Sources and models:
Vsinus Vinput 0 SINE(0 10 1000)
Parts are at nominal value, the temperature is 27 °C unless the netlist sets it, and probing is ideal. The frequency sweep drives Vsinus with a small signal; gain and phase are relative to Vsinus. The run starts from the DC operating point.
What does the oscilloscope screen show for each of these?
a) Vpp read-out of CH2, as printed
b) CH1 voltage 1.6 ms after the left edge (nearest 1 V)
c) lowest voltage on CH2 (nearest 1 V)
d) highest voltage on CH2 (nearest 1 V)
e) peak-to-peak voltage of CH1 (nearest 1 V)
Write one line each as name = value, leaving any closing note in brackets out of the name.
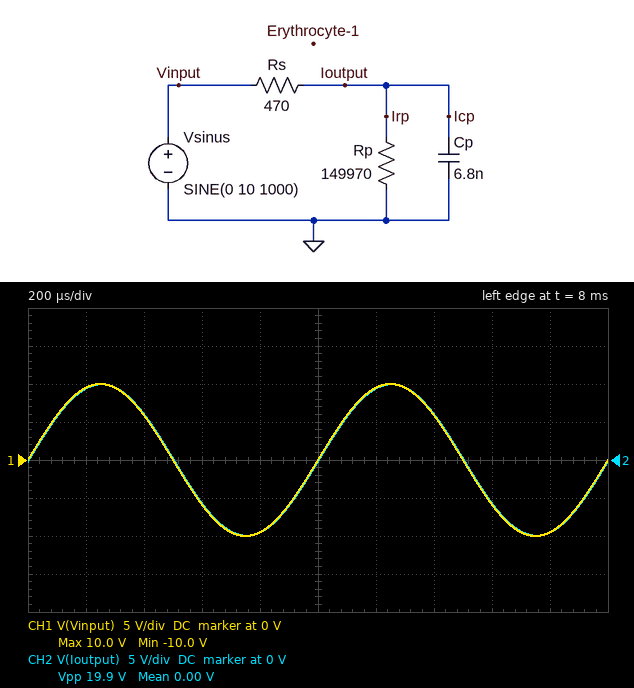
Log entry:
Vpp read-out of CH2, as printed = 19.9 V
CH1 voltage 1.6 ms after the left edge = -6 V
lowest voltage on CH2 = -10 V
highest voltage on CH2 = 10 V
peak-to-peak voltage of CH1 = 20 V
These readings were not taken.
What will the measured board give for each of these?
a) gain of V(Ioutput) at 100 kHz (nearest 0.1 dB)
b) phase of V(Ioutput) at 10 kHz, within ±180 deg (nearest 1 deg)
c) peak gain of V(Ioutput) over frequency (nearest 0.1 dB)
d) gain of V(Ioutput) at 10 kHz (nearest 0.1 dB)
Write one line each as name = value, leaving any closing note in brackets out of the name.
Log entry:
gain of V(Ioutput) at 100 kHz = -7.0 dB
phase of V(Ioutput) at 10 kHz, within ±180 deg = -11 deg
peak gain of V(Ioutput) over frequency = 0 dB
gain of V(Ioutput) at 10 kHz = -0.2 dB
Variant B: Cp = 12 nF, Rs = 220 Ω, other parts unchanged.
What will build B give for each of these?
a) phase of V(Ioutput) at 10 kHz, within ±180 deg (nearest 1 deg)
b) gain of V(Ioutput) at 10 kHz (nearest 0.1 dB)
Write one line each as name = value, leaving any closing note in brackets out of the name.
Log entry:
phase of V(Ioutput) at 10 kHz, within ±180 deg = -9 deg
gain of V(Ioutput) at 10 kHz = -0.1 dB
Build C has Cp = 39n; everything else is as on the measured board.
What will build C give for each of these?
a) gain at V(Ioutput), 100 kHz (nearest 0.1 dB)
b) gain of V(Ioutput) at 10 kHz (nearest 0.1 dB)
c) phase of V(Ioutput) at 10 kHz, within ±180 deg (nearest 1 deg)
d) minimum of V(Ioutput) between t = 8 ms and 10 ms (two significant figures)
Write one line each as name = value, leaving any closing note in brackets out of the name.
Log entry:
gain at V(Ioutput), 100 kHz = -21.3 dB
gain of V(Ioutput) at 10 kHz = -3.7 dB
phase of V(Ioutput) at 10 kHz, within ±180 deg = -49 deg
minimum of V(Ioutput) between t = 8 ms and 10 ms = -9.9 V
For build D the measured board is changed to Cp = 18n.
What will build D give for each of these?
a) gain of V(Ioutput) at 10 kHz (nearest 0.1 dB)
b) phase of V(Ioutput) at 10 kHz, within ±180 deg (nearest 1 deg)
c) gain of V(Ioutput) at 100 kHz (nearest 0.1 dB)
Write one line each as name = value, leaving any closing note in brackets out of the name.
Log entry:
gain of V(Ioutput) at 10 kHz = -1.1 dB
phase of V(Ioutput) at 10 kHz, within ±180 deg = -28 deg
gain of V(Ioutput) at 100 kHz = -14.7 dB
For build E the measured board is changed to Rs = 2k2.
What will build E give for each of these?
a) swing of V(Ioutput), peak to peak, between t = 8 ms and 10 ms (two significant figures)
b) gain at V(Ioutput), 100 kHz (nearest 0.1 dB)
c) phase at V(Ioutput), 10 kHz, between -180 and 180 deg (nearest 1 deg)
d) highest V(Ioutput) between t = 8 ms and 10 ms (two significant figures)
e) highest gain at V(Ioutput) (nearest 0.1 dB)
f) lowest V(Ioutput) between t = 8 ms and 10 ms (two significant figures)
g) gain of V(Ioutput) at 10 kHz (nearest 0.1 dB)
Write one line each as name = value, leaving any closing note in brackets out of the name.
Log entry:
swing of V(Ioutput), peak to peak, between t = 8 ms and 10 ms = 20 V
gain at V(Ioutput), 100 kHz = -19.5 dB
phase at V(Ioutput), 10 kHz, between -180 and 180 deg = -43 deg
highest V(Ioutput) between t = 8 ms and 10 ms = 9.8 V
highest gain at V(Ioutput) = -0.1 dB
lowest V(Ioutput) between t = 8 ms and 10 ms = -9.8 V
gain of V(Ioutput) at 10 kHz = -2.8 dB
